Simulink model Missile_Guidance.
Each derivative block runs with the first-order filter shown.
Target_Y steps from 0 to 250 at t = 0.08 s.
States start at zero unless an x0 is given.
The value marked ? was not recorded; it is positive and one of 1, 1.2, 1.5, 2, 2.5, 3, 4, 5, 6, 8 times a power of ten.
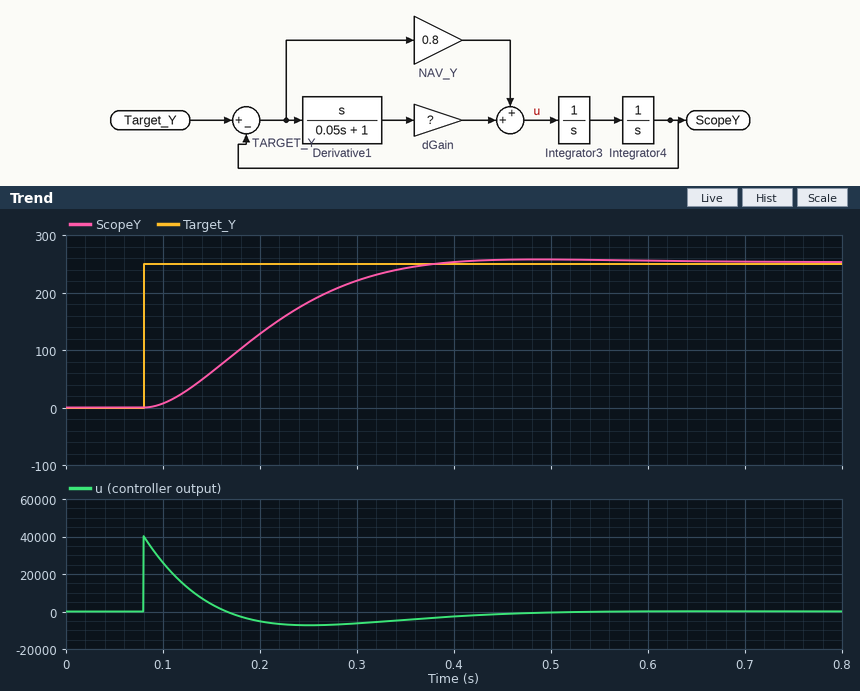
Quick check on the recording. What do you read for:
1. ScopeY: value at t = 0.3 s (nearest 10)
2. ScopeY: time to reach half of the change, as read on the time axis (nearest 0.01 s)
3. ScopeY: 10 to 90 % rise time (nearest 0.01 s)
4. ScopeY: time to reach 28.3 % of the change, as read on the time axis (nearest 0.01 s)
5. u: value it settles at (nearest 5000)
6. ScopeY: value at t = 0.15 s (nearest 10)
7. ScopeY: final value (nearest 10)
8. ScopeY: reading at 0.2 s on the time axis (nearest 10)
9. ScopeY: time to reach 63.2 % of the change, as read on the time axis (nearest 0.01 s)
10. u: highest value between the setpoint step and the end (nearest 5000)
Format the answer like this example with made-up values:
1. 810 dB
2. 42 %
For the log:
1. 220
2. 0.20 s
3. 0.19 s
4. 0.16 s
5. 0
6. 60
7. 250
8. 130
9. 0.23 s
10. 40000
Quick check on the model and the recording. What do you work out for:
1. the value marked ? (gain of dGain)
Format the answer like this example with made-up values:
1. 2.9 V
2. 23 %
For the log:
1. 8
